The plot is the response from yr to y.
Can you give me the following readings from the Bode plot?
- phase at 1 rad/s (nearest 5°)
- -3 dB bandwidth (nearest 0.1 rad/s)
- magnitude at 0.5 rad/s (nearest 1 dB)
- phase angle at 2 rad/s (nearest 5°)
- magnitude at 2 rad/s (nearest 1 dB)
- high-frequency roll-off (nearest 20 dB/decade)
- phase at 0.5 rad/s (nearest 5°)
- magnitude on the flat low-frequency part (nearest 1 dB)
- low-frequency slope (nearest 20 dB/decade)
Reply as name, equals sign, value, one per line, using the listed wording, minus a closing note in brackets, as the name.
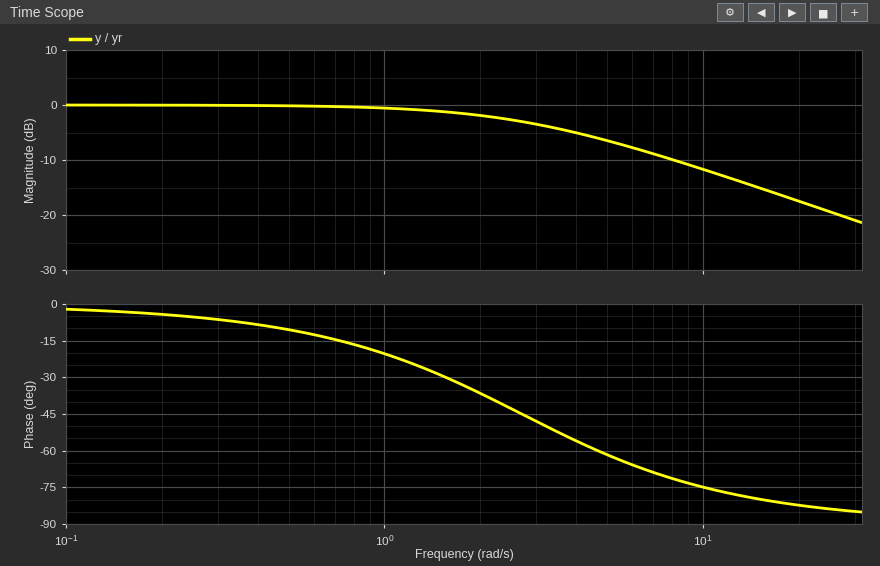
phase at 1 rad/s = -20°
-3 dB bandwidth = 2.7 rad/s
magnitude at 0.5 rad/s = 0 dB
phase angle at 2 rad/s = -35°
magnitude at 2 rad/s = -2 dB
high-frequency roll-off = -20 dB/decade
phase at 0.5 rad/s = -10°
magnitude on the flat low-frequency part = 0 dB
low-frequency slope = 0 dB/decade
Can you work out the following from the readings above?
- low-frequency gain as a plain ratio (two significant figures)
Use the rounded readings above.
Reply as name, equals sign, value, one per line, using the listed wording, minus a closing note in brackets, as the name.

low-frequency gain as a plain ratio = 1.0
